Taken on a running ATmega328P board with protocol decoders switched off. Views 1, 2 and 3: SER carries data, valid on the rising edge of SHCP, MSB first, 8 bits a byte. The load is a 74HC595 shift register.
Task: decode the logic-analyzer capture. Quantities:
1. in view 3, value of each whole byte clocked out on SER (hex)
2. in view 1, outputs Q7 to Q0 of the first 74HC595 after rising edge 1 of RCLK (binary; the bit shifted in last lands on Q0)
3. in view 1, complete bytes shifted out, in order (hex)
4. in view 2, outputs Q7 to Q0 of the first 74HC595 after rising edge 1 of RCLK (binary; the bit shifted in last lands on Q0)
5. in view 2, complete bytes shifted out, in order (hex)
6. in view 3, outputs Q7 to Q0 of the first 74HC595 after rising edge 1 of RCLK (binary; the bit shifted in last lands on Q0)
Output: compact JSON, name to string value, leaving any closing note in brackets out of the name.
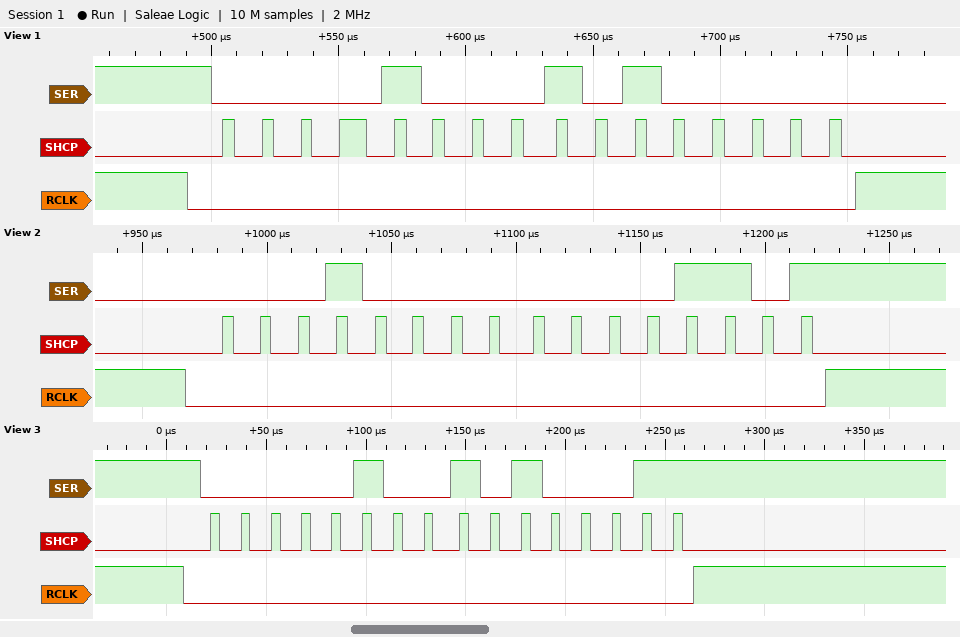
{"in view 3, value of each whole byte clocked out on SER": "04 A3", "in view 1, outputs Q7 to Q0 of the first 74HC595 after rising edge 1 of RCLK": "10100000", "in view 1, complete bytes shifted out, in order": "08 A0", "in view 2, outputs Q7 to Q0 of the first 74HC595 after rising edge 1 of RCLK": "00001101", "in view 2, complete bytes shifted out, in order": "10 0D", "in view 3, outputs Q7 to Q0 of the first 74HC595 after rising edge 1 of RCLK": "10100011"}
